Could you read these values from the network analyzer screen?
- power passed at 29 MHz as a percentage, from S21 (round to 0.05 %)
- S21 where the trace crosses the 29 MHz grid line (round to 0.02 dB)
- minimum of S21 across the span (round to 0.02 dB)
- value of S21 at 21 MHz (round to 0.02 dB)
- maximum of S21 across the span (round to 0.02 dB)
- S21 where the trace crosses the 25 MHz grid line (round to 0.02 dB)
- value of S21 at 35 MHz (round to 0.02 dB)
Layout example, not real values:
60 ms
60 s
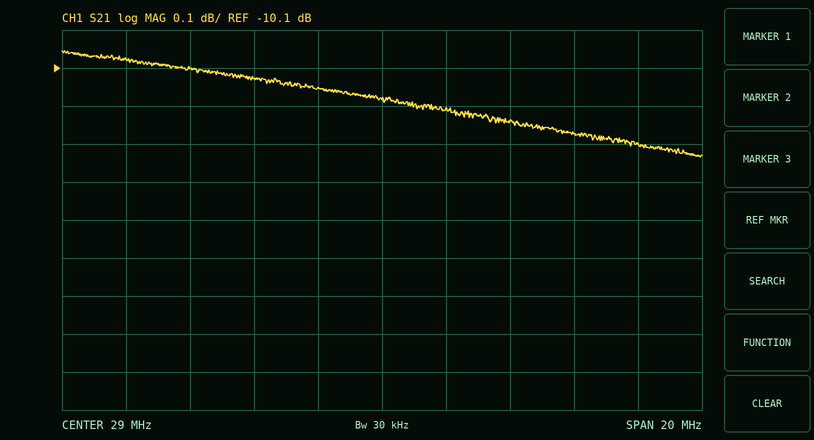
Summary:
9.60 %
-10.18 dB
-10.34 dB
-10.08 dB
-10.06 dB
-10.12 dB
-10.28 dB
